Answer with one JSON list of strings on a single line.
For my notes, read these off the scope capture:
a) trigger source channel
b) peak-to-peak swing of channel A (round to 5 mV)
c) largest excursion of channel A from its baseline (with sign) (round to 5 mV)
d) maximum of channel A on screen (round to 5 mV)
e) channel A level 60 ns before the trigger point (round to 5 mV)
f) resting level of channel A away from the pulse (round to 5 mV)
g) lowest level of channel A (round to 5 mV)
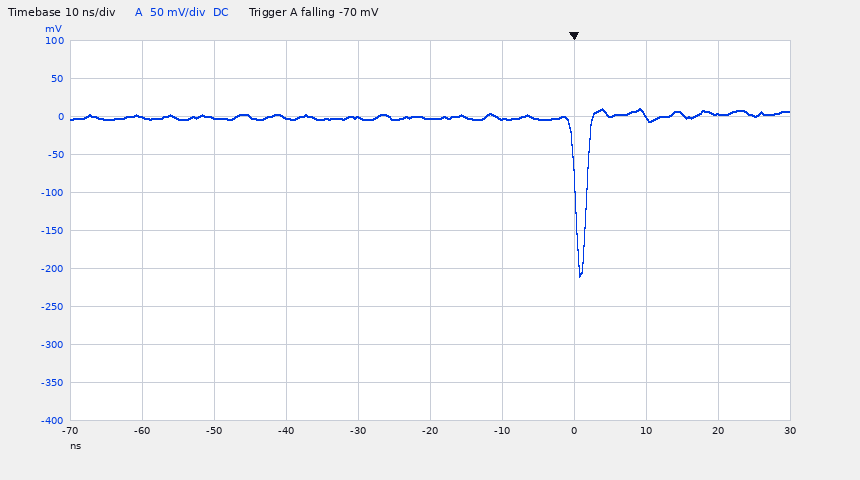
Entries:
["channel A", "220 mV", "-210 mV", "10 mV", "0 mV", "0 mV", "-210 mV"]
